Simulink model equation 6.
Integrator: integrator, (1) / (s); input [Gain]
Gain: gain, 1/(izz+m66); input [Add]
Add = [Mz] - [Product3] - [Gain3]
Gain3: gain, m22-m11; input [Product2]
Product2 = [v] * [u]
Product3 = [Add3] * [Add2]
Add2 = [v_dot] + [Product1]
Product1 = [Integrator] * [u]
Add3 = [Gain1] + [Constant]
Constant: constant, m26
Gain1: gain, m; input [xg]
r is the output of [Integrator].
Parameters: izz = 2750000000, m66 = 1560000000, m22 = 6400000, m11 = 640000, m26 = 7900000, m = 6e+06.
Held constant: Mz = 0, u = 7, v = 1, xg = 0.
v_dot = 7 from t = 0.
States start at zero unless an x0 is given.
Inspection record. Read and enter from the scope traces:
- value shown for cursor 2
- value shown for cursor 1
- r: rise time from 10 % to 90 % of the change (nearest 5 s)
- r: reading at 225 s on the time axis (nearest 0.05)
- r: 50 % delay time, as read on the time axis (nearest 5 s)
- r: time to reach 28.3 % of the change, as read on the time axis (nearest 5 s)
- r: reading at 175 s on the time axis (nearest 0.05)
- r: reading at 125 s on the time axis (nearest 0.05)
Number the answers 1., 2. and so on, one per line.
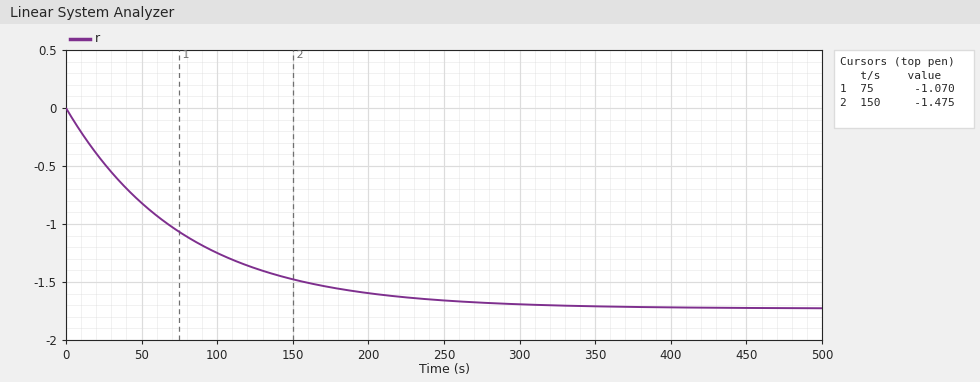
1. -1.475
2. -1.070
3. 170 s
4. -1.65
5. 55 s
6. 25 s
7. -1.55
8. -1.40
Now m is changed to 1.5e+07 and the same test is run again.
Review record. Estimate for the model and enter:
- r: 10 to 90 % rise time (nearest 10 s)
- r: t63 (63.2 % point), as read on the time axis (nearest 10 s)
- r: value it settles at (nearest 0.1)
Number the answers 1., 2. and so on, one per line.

1. 170 s
2. 80 s
3. -1.7
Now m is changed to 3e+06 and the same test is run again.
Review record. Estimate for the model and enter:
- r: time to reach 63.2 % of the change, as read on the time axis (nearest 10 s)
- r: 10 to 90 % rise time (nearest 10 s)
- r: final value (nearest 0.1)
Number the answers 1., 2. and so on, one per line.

1. 80 s
2. 170 s
3. -1.7
